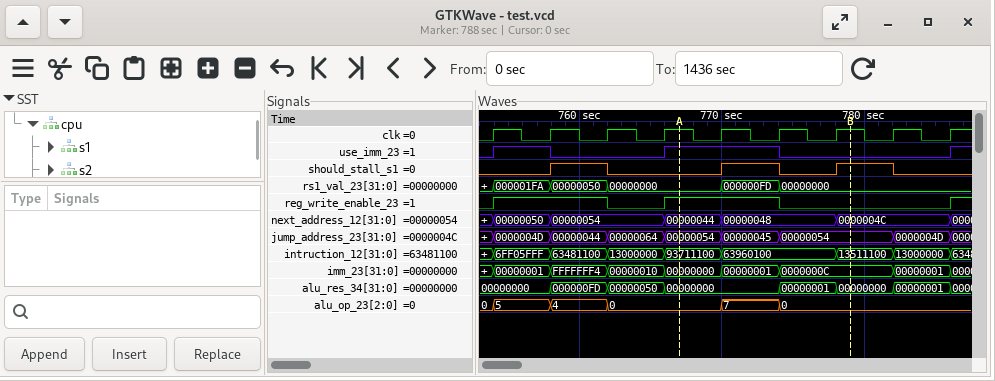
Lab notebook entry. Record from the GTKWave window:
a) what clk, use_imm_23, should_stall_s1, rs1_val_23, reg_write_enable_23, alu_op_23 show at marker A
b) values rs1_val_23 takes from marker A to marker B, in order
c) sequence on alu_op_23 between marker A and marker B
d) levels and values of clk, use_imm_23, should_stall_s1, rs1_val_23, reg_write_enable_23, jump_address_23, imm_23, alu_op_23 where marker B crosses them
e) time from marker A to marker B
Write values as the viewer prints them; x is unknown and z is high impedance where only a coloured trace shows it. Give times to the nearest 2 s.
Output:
clk=1, use_imm_23=1, should_stall_s1=0, rs1_val_23=00000000, reg_write_enable_23=1, alu_op_23=0
00000000, 000000FD, 00000000
0, 7, 0
clk=1, use_imm_23=0, should_stall_s1=1, rs1_val_23=00000000, reg_write_enable_23=0, jump_address_23=00000054, imm_23=0000000C, alu_op_23=0
12 s
